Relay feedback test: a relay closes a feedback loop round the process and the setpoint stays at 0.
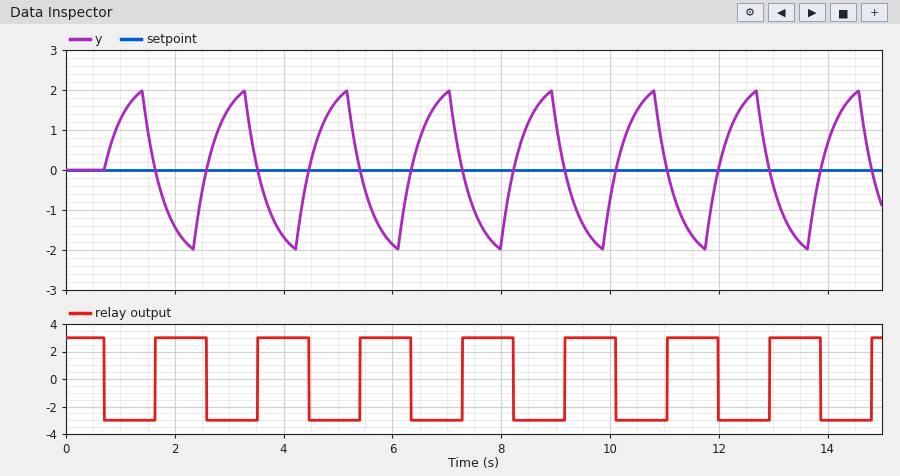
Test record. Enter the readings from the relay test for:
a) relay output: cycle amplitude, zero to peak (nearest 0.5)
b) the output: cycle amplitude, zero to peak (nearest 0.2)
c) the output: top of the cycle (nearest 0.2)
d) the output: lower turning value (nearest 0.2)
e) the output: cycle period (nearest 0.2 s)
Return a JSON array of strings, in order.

["3.0", "2.0", "2.0", "-2.0", "1.8 s"]
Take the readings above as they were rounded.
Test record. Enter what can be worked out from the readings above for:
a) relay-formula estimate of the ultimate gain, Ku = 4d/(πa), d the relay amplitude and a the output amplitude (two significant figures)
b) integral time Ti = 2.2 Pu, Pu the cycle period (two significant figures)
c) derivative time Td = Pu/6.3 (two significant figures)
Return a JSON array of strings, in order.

["1.9", "4.0 s", "0.29 s"]
